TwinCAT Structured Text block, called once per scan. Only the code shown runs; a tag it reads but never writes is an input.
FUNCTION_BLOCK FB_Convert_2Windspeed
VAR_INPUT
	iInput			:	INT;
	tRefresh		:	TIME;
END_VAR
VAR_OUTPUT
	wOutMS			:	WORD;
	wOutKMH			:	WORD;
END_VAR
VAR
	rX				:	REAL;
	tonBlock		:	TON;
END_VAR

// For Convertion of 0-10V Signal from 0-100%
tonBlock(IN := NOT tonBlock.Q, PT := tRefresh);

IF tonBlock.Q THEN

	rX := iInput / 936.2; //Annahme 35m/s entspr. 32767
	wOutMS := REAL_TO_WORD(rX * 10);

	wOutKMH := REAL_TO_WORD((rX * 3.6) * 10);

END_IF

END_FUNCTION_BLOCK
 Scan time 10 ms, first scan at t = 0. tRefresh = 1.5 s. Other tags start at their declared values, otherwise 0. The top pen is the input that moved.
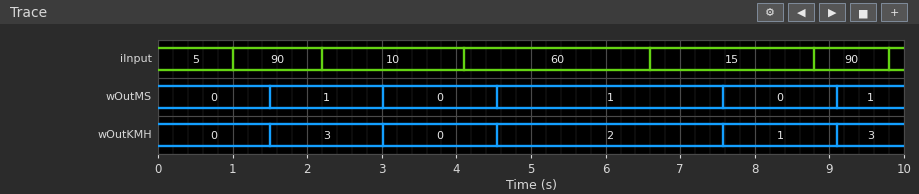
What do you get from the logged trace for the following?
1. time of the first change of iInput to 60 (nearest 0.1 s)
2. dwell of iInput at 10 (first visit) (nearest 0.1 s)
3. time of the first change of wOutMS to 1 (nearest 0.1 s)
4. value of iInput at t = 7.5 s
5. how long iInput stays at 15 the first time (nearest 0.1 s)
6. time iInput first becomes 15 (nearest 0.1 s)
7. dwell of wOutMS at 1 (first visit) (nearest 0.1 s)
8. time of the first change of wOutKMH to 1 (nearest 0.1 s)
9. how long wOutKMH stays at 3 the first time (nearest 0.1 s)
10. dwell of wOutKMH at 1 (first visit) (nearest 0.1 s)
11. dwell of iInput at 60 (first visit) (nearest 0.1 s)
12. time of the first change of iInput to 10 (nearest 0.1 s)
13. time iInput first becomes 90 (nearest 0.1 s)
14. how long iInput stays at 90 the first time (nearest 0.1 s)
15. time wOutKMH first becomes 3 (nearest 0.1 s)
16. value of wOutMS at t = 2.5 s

4.1 s
1.9 s
1.5 s
15
2.2 s
6.6 s
1.5 s
7.6 s
1.5 s
1.5 s
2.5 s
2.2 s
1.0 s
1.2 s
1.5 s
1
